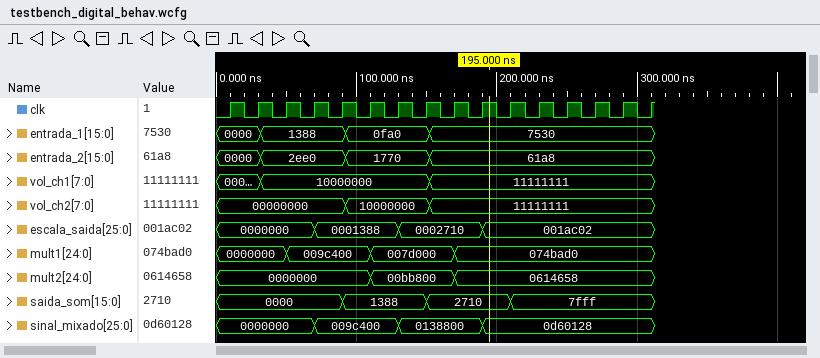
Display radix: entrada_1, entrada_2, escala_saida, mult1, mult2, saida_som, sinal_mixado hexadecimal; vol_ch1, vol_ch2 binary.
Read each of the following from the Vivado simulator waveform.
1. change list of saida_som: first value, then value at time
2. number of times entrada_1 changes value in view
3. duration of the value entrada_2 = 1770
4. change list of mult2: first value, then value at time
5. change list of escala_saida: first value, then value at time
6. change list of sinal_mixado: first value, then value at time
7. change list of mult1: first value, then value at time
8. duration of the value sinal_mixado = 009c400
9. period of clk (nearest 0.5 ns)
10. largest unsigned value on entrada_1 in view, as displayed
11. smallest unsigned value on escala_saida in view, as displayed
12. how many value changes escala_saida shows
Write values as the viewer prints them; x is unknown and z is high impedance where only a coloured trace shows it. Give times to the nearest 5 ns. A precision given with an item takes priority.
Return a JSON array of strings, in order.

["0000, 1388 at 90 ns, 2710 at 150 ns, 7fff at 210 ns", "3", "60 ns", "0000000, 00bb800 at 110 ns, 0614658 at 170 ns", "0000000, 0001388 at 70 ns, 0002710 at 130 ns, 001ac02 at 190 ns", "0000000, 009c400 at 70 ns, 0138800 at 130 ns, 0d60128 at 190 ns", "0000000, 009c400 at 50 ns, 007d000 at 110 ns, 074bad0 at 170 ns", "60 ns", "20 ns", "7530", "0000000", "3"]
